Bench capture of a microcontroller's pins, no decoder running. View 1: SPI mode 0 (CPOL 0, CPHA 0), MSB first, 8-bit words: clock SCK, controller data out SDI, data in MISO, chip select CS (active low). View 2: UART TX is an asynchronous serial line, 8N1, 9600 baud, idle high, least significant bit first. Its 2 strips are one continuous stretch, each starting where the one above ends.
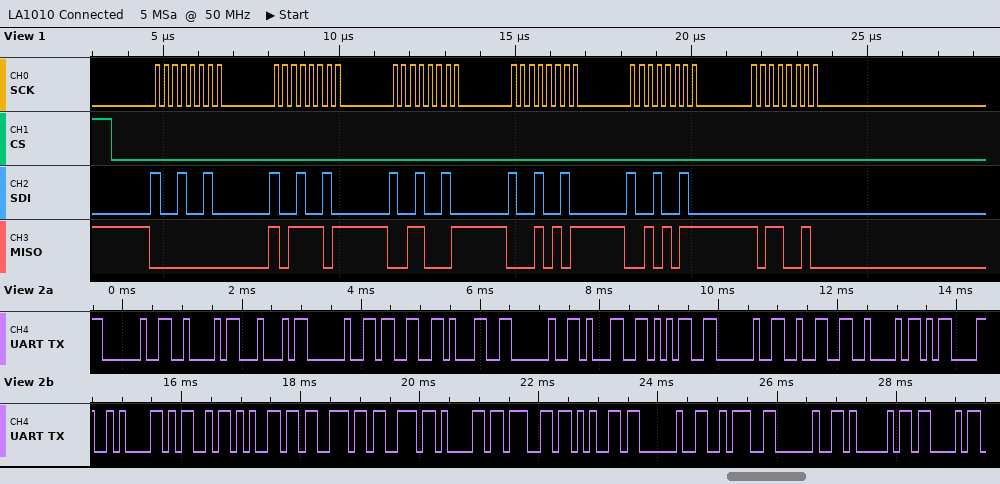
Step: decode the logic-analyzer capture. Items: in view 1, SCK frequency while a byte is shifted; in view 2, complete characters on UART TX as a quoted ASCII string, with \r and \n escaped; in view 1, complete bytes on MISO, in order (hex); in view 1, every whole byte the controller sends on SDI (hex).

4 MHz
" BD 31 15 2B\r\nMessage : AC"
0x00 0xBD 0x31 0x15 0x2B 0xB2
0x92 0x92 0x92 0x92 0x92 0x00
